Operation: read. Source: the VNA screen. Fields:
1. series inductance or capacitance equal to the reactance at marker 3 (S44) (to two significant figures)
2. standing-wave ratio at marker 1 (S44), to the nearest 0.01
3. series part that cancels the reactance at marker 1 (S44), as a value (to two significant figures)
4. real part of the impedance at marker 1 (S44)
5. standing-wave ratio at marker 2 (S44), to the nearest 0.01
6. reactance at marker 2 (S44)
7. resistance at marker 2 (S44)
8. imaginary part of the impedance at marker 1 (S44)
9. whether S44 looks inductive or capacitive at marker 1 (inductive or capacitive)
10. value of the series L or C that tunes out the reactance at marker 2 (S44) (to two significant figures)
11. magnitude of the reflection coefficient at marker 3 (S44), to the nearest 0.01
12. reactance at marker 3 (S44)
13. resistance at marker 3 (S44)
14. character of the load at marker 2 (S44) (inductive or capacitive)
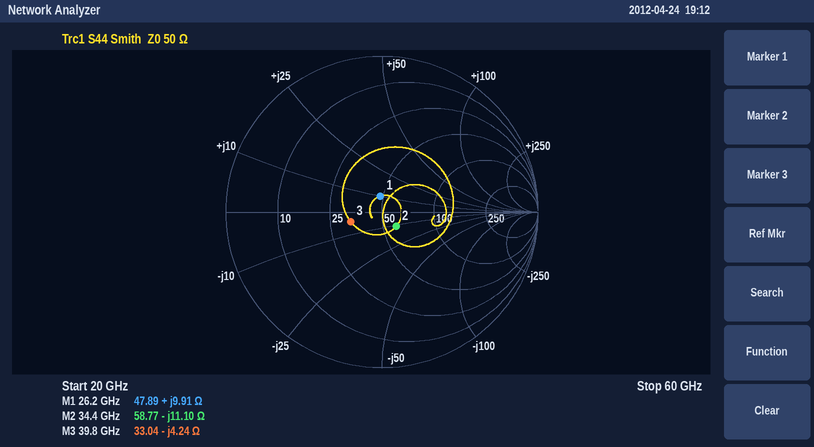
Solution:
940 fF
1.23
610 fF
47.89 Ω
1.30
-11.10 Ω
58.77 Ω
+9.91 Ω
inductive
51 pH
0.21
-4.24 Ω
33.04 Ω
capacitive
